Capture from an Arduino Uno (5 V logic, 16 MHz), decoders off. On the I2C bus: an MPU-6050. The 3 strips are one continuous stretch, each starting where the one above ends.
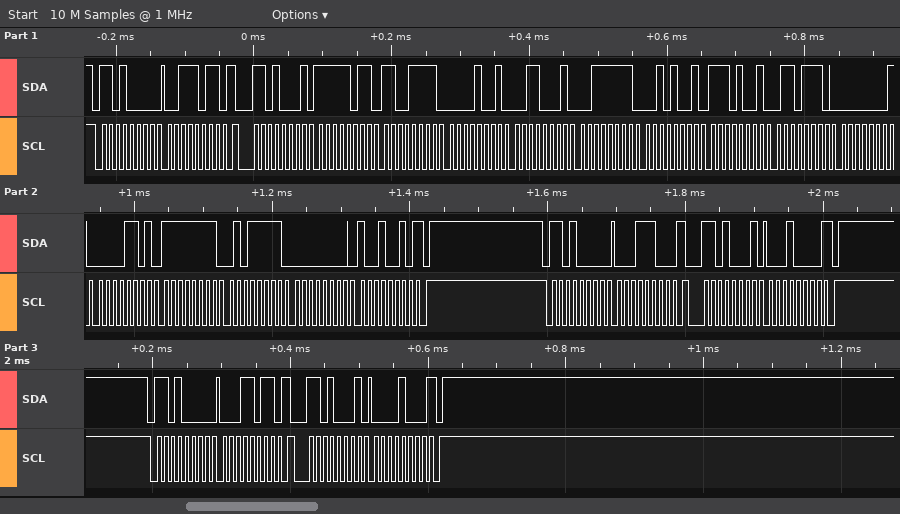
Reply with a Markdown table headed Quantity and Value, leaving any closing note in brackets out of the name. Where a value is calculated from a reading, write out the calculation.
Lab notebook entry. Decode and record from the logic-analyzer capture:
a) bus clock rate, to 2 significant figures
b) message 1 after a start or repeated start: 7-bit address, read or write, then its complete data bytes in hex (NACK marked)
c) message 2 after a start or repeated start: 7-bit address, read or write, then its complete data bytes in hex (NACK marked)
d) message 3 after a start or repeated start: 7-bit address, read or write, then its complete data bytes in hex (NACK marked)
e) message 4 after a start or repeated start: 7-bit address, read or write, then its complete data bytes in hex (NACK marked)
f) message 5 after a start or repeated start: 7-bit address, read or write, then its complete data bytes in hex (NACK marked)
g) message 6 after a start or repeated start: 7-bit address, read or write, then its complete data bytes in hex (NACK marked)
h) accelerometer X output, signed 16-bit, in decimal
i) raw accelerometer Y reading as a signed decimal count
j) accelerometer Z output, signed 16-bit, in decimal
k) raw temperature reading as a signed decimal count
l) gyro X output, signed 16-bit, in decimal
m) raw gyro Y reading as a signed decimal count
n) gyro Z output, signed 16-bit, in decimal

| Quantity | Value |
|---|---|
| bus clock rate, to 2 significant figures | 100 kHz |
| message 1 after a start or repeated start: 7-bit address, read or write, then its complete data bytes in hex | 0x68 write: 3B |
| message 2 after a start or repeated start: 7-bit address, read or write, then its complete data bytes in hex | 0x68 read: FB CF 09 31 3F 29 E9 6E 01 0D FF 5F 00 92 NACK |
| message 3 after a start or repeated start: 7-bit address, read or write, then its complete data bytes in hex | 0x68 write: 1C |
| message 4 after a start or repeated start: 7-bit address, read or write, then its complete data bytes in hex | 0x68 read: 10 NACK |
| message 5 after a start or repeated start: 7-bit address, read or write, then its complete data bytes in hex | 0x68 write: 1B |
| message 6 after a start or repeated start: 7-bit address, read or write, then its complete data bytes in hex | 0x68 read: 08 NACK |
| accelerometer X output, signed 16-bit, in decimal | 0xFBCF = -1073 |
| raw accelerometer Y reading as a signed decimal count | 0x0931 = 2353 |
| accelerometer Z output, signed 16-bit, in decimal | 0x3F29 = 16169 |
| raw temperature reading as a signed decimal count | 0xE96E = -5778 |
| gyro X output, signed 16-bit, in decimal | 0x010D = 269 |
| raw gyro Y reading as a signed decimal count | 0xFF5F = -161 |
| gyro Z output, signed 16-bit, in decimal | 0x0092 = 146 |
